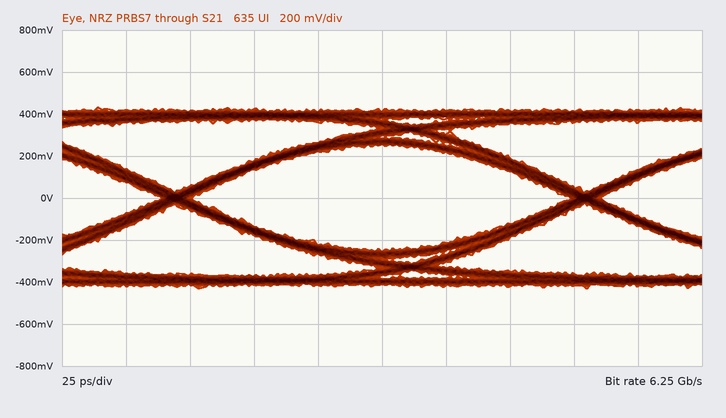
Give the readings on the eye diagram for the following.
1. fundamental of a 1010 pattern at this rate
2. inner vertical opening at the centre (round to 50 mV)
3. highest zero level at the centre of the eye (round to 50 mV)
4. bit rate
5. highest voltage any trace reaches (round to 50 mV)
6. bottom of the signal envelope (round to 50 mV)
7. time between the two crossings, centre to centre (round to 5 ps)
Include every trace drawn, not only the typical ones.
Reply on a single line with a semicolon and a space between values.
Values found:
3.125 GHz; 500 mV; -250 mV; 6.25 Gb/s; 450 mV; -450 mV; 160 ps
